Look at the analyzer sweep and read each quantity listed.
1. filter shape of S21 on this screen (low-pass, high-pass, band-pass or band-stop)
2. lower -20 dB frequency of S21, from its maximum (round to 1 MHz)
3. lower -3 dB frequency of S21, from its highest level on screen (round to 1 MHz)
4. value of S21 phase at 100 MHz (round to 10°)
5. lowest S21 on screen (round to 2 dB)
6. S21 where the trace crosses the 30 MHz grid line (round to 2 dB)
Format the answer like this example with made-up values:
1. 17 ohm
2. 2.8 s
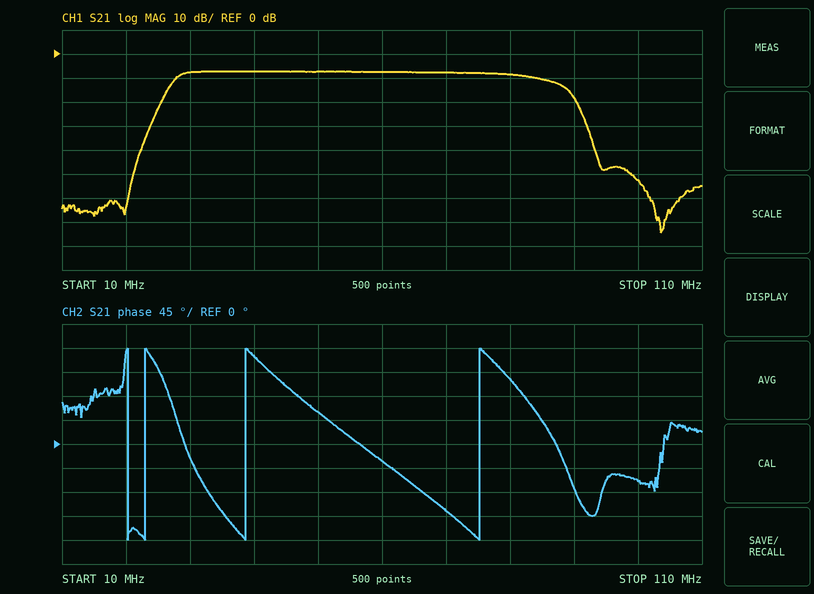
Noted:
1. band-pass
2. 24 MHz
3. 28 MHz
4. -70°
5. -74 dB
6. -8 dB
